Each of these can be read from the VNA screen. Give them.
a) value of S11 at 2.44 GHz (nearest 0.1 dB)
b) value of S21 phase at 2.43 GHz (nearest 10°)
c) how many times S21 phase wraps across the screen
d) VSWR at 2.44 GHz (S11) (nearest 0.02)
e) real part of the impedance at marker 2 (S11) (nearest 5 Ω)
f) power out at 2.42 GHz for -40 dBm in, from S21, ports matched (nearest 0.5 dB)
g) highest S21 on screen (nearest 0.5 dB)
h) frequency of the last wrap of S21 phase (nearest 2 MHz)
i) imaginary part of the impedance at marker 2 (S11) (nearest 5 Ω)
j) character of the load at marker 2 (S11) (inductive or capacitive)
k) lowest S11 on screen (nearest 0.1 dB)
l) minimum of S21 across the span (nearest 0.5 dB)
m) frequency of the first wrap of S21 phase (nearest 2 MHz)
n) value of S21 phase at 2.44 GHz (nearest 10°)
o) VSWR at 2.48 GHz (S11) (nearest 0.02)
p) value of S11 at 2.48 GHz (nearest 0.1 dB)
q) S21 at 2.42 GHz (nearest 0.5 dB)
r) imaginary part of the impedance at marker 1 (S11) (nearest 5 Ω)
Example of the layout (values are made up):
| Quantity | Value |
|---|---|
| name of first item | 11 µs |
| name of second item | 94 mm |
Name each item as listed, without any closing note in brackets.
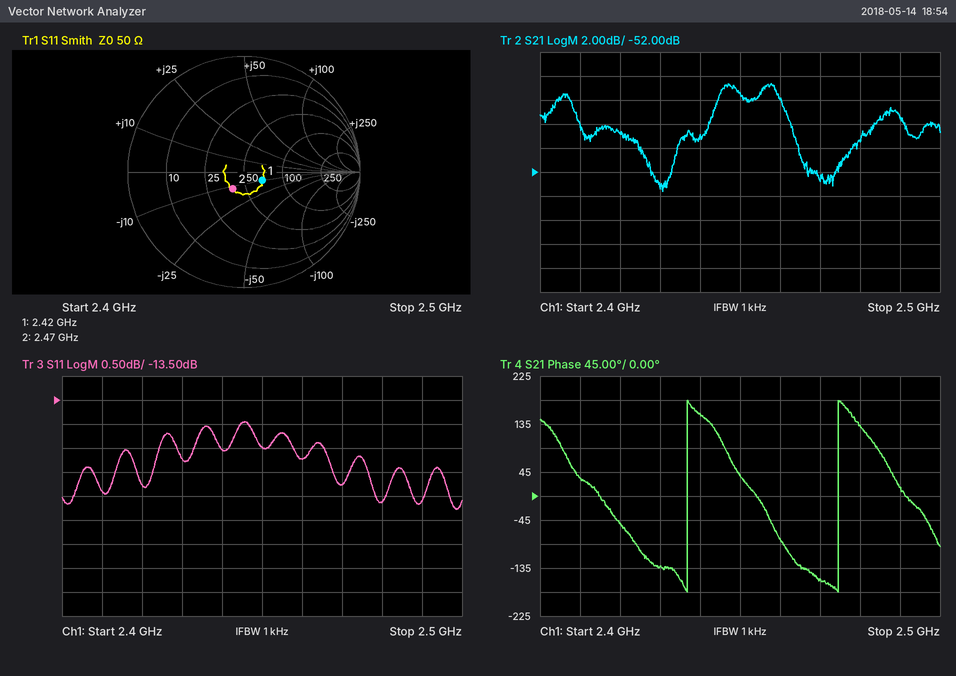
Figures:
| Quantity | Value |
|---|---|
| value of S11 at 2.44 GHz | -14.5 dB |
| value of S21 phase at 2.43 GHz | -130° |
| how many times S21 phase wraps across the screen | 2 |
| VSWR at 2.44 GHz (S11) | 1.46 |
| real part of the impedance at marker 2 (S11) | 40 Ω |
| power out at 2.42 GHz for -40 dBm in, from S21, ports matched | -89.0 dBm |
| highest S21 on screen | -44.5 dB |
| frequency of the last wrap of S21 phase | 2.474 GHz |
| imaginary part of the impedance at marker 2 (S11) | -10 Ω |
| character of the load at marker 2 (S11) | capacitive |
| lowest S11 on screen | -15.8 dB |
| minimum of S21 across the span | -53.5 dB |
| frequency of the first wrap of S21 phase | 2.436 GHz |
| value of S21 phase at 2.44 GHz | 150° |
| VSWR at 2.48 GHz (S11) | 1.40 |
| value of S11 at 2.48 GHz | -15.6 dB |
| S21 at 2.42 GHz | -49.0 dB |
| imaginary part of the impedance at marker 1 (S11) | -10 Ω |
